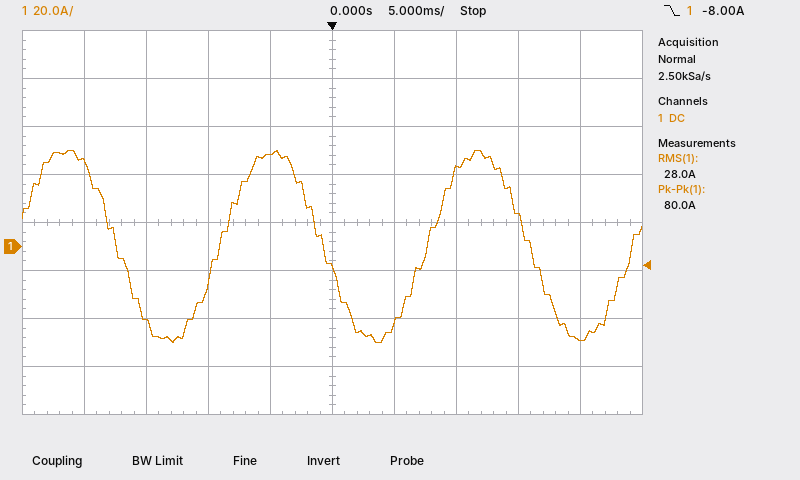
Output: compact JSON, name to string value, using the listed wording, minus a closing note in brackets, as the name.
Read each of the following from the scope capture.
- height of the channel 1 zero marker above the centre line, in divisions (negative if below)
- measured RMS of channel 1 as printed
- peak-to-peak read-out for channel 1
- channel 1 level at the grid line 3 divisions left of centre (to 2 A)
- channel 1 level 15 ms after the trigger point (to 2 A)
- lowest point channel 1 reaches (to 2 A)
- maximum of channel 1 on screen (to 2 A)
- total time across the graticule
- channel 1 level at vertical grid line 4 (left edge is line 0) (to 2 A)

{"height of the channel 1 zero marker above the centre line, in divisions": "-0.5 div", "measured RMS of channel 1 as printed": "28.0 A", "peak-to-peak read-out for channel 1": "80.0 A", "channel 1 level at the grid line 3 divisions left of centre": "-32 A", "channel 1 level 15 ms after the trigger point": "12 A", "lowest point channel 1 reaches": "-40 A", "maximum of channel 1 on screen": "40 A", "total time across the graticule": "50 ms", "channel 1 level at vertical grid line 4 (left edge is line 0)": "38 A"}
